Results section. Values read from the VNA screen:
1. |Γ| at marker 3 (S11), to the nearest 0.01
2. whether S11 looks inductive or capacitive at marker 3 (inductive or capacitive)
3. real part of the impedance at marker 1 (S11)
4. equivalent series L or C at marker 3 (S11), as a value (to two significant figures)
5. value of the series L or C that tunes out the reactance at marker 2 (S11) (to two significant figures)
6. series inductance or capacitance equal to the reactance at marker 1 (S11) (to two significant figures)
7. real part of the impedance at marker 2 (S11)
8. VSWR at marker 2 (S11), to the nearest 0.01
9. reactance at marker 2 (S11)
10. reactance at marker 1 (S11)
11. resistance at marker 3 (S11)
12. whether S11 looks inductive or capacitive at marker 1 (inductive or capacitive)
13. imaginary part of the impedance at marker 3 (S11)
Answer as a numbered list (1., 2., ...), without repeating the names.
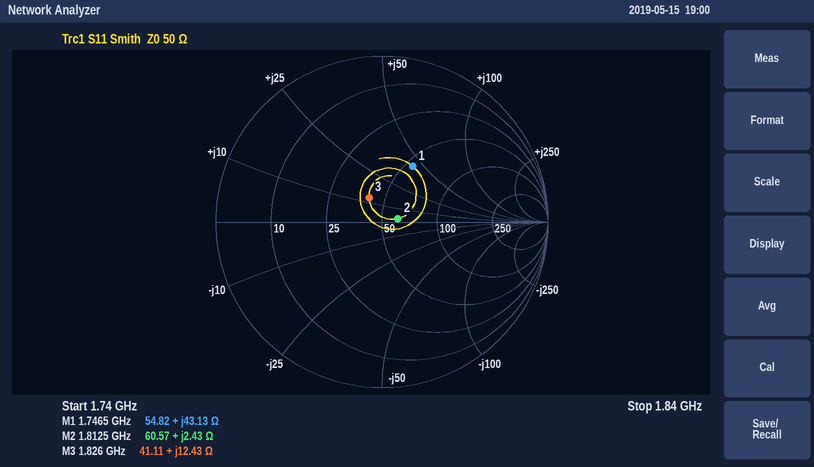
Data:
1. 0.17
2. inductive
3. 54.82 Ω
4. 1.1 nH
5. 36 pF
6. 3.9 nH
7. 60.57 Ω
8. 1.22
9. +2.43 Ω
10. +43.13 Ω
11. 41.11 Ω
12. inductive
13. +12.43 Ω
